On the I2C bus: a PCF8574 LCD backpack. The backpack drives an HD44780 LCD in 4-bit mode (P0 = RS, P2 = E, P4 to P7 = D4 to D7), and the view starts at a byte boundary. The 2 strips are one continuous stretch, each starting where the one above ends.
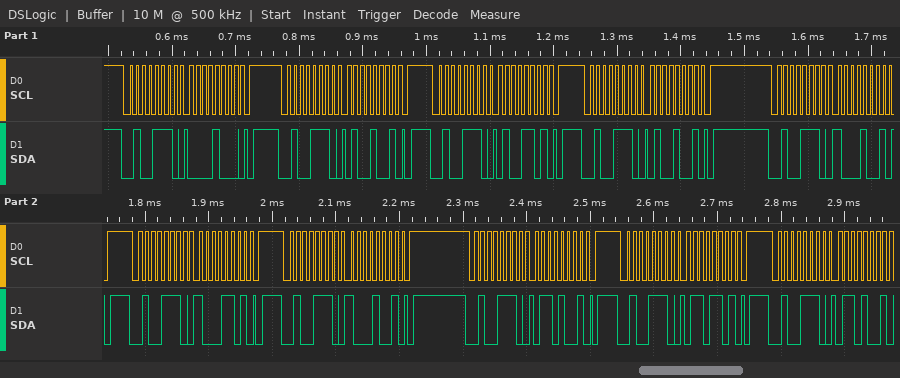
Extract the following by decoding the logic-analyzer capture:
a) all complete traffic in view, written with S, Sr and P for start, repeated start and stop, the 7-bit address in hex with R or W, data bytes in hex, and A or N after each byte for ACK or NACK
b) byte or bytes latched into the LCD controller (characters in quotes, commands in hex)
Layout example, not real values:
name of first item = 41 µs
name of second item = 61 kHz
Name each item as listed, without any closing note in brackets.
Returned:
all complete traffic in view, written with S, Sr and P for start, repeated start and stop, the 7-bit address in hex with R or W, data bytes in hex, and A or N after each byte for ACK or NACK = S 27W A 08 A P S 27W A 49 A P S 27W A 4D A P S 27W A 49 A P S 27W A 89 A P S 27W A 8D A P S 27W A 89 A P S 27W A 69 A P S 27W A 6D A P S 27W A 69 A
byte or bytes latched into the LCD controller = 'H'
